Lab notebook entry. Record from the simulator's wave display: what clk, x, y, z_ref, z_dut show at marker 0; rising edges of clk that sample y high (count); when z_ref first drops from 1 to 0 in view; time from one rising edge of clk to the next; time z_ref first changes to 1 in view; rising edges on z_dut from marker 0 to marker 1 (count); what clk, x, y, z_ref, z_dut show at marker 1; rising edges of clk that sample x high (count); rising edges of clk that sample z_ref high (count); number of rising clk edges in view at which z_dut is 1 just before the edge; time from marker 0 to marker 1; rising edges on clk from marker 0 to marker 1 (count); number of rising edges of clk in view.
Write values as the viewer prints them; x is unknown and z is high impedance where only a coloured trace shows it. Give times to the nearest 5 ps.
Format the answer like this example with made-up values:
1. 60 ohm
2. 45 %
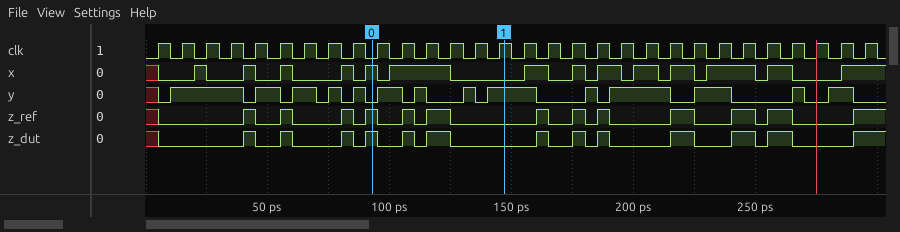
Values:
1. clk=0, x=1, y=0, z_ref=1, z_dut=1
2. 16
3. 45 ps
4. 10 ps
5. 40 ps
6. 2
7. clk=1, x=0, y=1, z_ref=0, z_dut=0
8. 15
9. 9
10. 9
11. 55 ps
12. 6
13. 30
